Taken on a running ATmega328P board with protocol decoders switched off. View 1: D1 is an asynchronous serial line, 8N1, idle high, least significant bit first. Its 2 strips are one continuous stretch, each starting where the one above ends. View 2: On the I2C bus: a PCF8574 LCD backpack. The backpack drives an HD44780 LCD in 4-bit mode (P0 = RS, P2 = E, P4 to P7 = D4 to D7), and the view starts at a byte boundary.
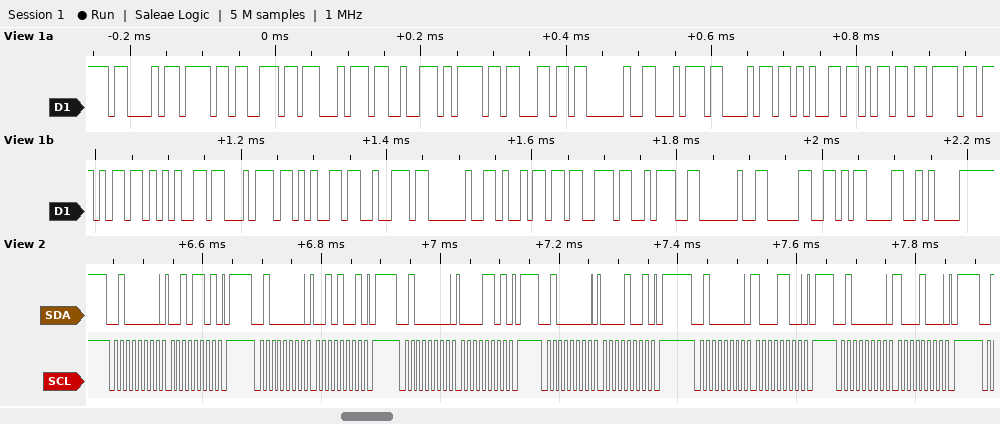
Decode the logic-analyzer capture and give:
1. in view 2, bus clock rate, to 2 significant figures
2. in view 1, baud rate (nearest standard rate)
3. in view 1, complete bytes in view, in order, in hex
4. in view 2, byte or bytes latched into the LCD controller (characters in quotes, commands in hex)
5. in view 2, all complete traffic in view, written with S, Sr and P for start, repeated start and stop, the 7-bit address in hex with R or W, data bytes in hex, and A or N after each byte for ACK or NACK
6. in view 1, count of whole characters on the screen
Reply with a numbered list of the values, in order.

1. 100 kHz
2. 115200 baud
3. 43 6F 6E 74 72 6F 6C 20 74 68 65 6D 6F 6D 65 74 65 72 20 69 73 3A 20 30 0D 0A
4. ' '
5. S 20W A 2D A P S 20W A 29 A P S 20W A 0D A P S 20W A 09 A P S 20W A 8C A P S 20W A 88 A P
6. 26
